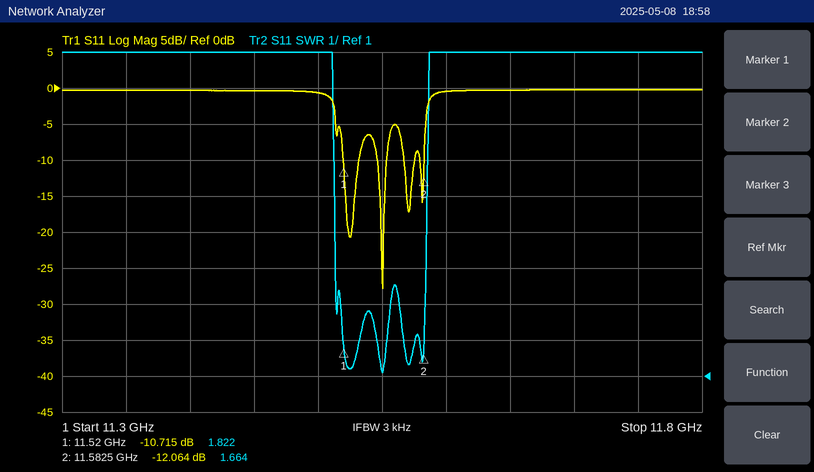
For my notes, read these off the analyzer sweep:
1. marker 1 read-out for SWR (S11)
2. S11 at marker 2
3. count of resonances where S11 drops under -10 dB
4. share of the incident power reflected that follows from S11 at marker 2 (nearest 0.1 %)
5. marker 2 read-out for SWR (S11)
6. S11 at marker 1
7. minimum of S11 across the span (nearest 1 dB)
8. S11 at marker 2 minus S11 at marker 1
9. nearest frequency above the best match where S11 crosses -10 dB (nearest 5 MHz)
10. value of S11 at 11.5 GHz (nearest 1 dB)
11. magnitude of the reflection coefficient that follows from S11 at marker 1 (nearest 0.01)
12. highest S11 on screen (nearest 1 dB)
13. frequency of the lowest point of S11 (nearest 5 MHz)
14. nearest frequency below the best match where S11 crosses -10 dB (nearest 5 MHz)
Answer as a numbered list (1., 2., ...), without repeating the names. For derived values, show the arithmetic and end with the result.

1. 1.822
2. -12.064 dB
3. 4
4. 10^(-12.064/10) ≈ 6.2 %
5. 1.664
6. -10.715 dB
7. -28 dB
8. -12.064 − (-10.715) = -1.349 dB
9. 11.555 GHz
10. -1 dB
11. 10^(-10.715/20) ≈ 0.29
12. 0 dB
13. 11.550 GHz
14. 11.545 GHz
